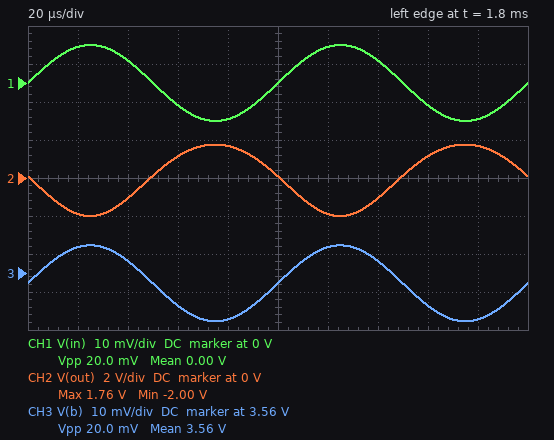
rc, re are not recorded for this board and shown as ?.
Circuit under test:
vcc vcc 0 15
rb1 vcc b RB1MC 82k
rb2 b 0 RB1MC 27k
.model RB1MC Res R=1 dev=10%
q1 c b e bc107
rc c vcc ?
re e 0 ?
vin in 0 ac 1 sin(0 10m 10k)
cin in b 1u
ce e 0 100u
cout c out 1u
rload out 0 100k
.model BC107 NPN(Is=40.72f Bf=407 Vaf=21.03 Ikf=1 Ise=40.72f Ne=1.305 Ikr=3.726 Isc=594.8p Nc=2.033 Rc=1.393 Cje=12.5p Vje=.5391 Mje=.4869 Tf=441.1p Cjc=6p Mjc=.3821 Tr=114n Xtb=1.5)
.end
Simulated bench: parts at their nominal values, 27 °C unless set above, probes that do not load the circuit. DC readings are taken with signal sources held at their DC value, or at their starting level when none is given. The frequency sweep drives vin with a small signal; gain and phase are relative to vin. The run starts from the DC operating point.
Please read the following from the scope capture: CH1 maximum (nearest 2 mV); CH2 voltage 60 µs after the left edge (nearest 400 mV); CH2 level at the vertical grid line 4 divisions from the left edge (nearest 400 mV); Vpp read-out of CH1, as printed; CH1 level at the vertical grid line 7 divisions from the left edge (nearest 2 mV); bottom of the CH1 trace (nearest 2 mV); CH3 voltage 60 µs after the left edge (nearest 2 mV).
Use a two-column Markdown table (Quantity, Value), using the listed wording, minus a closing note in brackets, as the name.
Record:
| Quantity | Value |
|---|---|
| CH1 maximum | 10 mV |
| CH2 voltage 60 µs after the left edge | 1.2 V |
| CH2 level at the vertical grid line 4 divisions from the left edge | 1.6 V |
| Vpp read-out of CH1, as printed | 20.0 mV |
| CH1 level at the vertical grid line 7 divisions from the left edge | 6 mV |
| bottom of the CH1 trace | -10 mV |
| CH3 voltage 60 µs after the left edge | 3.552 V |
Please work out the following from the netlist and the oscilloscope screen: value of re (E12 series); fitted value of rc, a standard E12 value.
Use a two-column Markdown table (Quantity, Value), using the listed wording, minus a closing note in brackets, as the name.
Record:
| Quantity | Value |
|---|---|
| value of re | 1.8 kΩ |
| fitted value of rc, a standard E12 value | 3.9 kΩ |
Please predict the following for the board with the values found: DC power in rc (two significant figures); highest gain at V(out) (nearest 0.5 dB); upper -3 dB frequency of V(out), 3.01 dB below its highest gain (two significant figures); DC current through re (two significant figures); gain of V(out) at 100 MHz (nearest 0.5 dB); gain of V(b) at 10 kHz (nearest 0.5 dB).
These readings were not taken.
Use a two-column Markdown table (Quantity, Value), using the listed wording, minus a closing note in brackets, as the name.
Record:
| Quantity | Value |
|---|---|
| DC power in rc | 10 mW |
| highest gain at V(out) | 45.5 dB |
| upper -3 dB frequency of V(out), 3.01 dB below its highest gain | 19 MHz |
| DC current through re | 1.6 mA |
| gain of V(out) at 100 MHz | 31.0 dB |
| gain of V(b) at 10 kHz | 0 dB |
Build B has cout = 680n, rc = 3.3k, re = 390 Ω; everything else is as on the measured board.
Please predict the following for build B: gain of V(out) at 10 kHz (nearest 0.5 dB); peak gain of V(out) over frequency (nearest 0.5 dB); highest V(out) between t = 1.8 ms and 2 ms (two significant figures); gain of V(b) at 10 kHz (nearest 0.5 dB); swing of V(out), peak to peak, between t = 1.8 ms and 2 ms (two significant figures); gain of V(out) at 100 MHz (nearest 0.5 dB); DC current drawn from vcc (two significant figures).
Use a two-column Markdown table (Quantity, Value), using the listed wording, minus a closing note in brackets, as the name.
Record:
| Quantity | Value |
|---|---|
| gain of V(out) at 10 kHz | 29.0 dB |
| peak gain of V(out) over frequency | 33.0 dB |
| highest V(out) between t = 1.8 ms and 2 ms | 4.2 V |
| gain of V(b) at 10 kHz | -4.0 dB |
| swing of V(out), peak to peak, between t = 1.8 ms and 2 ms | 4.3 V |
| gain of V(out) at 100 MHz | 5.0 dB |
| DC current drawn from vcc | 4.2 mA |
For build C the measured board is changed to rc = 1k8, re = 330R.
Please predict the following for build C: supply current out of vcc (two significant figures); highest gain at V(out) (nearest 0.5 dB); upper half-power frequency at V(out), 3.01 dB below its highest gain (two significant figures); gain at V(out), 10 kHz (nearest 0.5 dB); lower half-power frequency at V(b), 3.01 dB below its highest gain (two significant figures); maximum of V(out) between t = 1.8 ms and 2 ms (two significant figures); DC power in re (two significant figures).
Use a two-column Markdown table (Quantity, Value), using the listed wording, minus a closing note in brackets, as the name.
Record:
| Quantity | Value |
|---|---|
| supply current out of vcc | 7.1 mA |
| highest gain at V(out) | 48.5 dB |
| upper half-power frequency at V(out), 3.01 dB below its highest gain | 14 MHz |
| gain at V(out), 10 kHz | 48.0 dB |
| lower half-power frequency at V(b), 3.01 dB below its highest gain | 3.2 kHz |
| maximum of V(out) between t = 1.8 ms and 2 ms | 4.6 V |
| DC power in re | 16 mW |
